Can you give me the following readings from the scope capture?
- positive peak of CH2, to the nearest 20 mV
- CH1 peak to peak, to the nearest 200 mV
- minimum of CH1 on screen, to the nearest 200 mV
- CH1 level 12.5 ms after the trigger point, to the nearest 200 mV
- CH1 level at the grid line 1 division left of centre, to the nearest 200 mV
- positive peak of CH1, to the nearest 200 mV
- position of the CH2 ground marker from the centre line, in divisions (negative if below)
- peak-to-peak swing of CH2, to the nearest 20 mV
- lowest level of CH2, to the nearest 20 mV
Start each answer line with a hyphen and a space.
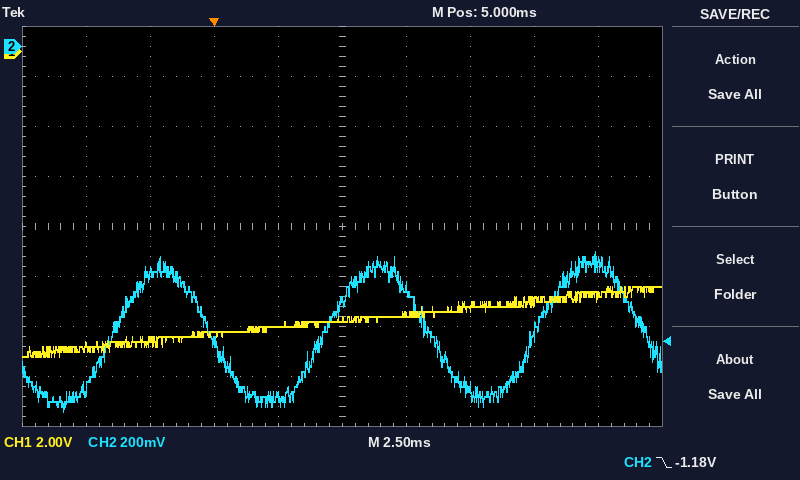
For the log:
- -820 mV
- 2.8 V
- -12.2 V
- -10.0 V
- -11.0 V
- -9.4 V
- +3.6 div
- 640 mV
- -1.46 V
